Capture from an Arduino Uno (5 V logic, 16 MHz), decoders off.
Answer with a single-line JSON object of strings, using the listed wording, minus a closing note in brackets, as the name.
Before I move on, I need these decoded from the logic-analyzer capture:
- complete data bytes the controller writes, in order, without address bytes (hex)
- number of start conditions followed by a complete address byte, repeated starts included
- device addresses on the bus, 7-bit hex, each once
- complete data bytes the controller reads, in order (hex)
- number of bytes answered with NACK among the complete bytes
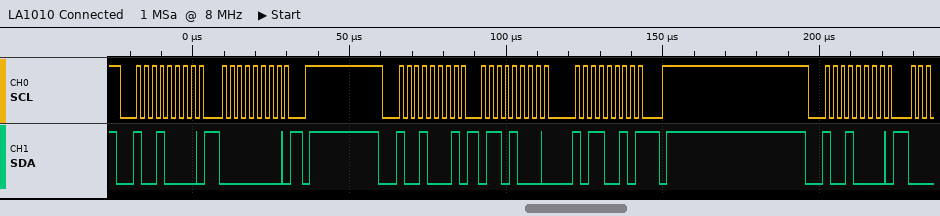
{"complete data bytes the controller writes, in order, without address bytes": "00", "number of start conditions followed by a complete address byte, repeated starts included": "3", "device addresses on the bus, 7-bit hex, each once": "0x48", "complete data bytes the controller reads, in order": "68 B2", "number of bytes answered with NACK among the complete bytes": "1"}
